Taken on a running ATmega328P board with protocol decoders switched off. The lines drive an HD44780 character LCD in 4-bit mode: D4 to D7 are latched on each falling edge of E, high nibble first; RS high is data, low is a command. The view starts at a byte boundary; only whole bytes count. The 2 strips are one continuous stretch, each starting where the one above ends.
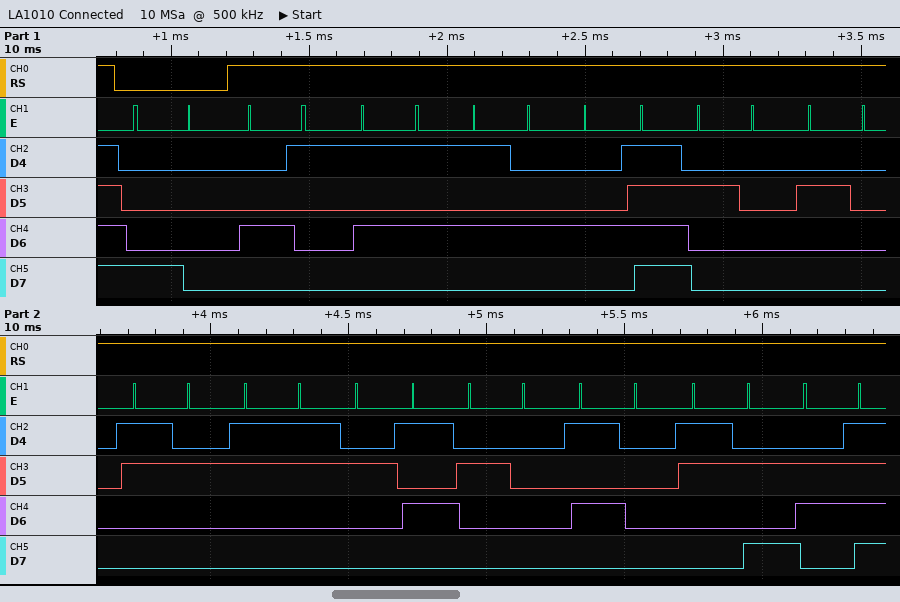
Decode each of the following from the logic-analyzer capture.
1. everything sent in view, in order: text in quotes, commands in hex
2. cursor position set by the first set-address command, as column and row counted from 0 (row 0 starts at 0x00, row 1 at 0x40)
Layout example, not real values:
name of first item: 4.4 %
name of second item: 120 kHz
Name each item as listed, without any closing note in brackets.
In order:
everything sent in view, in order: text in quotes, commands in hex: 0x80 "AUTO  23% P:o"
cursor position set by the first set-address command, as column and row counted from 0: column 0, row 0
